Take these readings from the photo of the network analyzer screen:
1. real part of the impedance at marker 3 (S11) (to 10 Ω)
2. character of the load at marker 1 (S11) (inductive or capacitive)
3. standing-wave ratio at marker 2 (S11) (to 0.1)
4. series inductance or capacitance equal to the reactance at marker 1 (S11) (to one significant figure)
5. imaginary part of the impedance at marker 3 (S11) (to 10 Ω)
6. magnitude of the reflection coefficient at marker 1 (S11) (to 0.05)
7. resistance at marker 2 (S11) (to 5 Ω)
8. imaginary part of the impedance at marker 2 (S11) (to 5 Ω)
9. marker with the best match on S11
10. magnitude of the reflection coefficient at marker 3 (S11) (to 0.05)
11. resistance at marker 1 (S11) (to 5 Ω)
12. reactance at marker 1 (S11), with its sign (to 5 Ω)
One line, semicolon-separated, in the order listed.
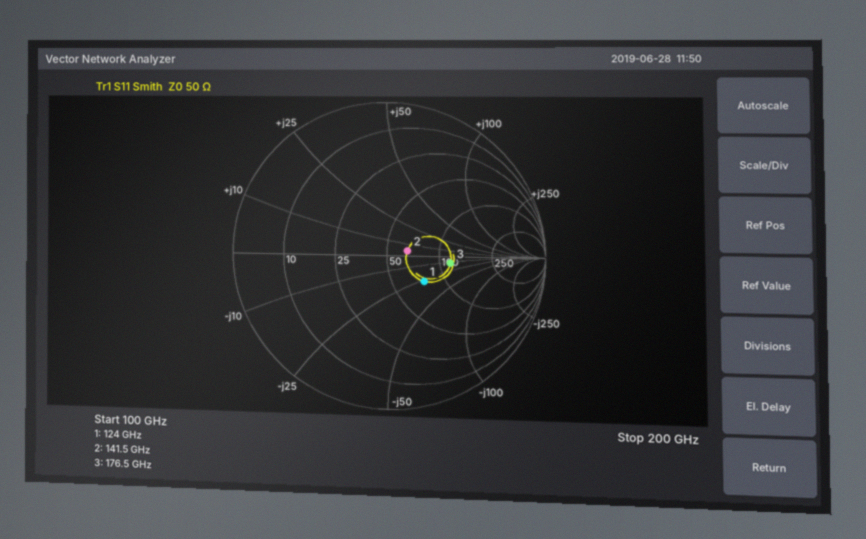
120 Ω; capacitive; 1.3; 50 fF; -10 Ω; 0.30; 65 Ω; +5 Ω; marker 2; 0.40; 75 Ω; -25 Ω
